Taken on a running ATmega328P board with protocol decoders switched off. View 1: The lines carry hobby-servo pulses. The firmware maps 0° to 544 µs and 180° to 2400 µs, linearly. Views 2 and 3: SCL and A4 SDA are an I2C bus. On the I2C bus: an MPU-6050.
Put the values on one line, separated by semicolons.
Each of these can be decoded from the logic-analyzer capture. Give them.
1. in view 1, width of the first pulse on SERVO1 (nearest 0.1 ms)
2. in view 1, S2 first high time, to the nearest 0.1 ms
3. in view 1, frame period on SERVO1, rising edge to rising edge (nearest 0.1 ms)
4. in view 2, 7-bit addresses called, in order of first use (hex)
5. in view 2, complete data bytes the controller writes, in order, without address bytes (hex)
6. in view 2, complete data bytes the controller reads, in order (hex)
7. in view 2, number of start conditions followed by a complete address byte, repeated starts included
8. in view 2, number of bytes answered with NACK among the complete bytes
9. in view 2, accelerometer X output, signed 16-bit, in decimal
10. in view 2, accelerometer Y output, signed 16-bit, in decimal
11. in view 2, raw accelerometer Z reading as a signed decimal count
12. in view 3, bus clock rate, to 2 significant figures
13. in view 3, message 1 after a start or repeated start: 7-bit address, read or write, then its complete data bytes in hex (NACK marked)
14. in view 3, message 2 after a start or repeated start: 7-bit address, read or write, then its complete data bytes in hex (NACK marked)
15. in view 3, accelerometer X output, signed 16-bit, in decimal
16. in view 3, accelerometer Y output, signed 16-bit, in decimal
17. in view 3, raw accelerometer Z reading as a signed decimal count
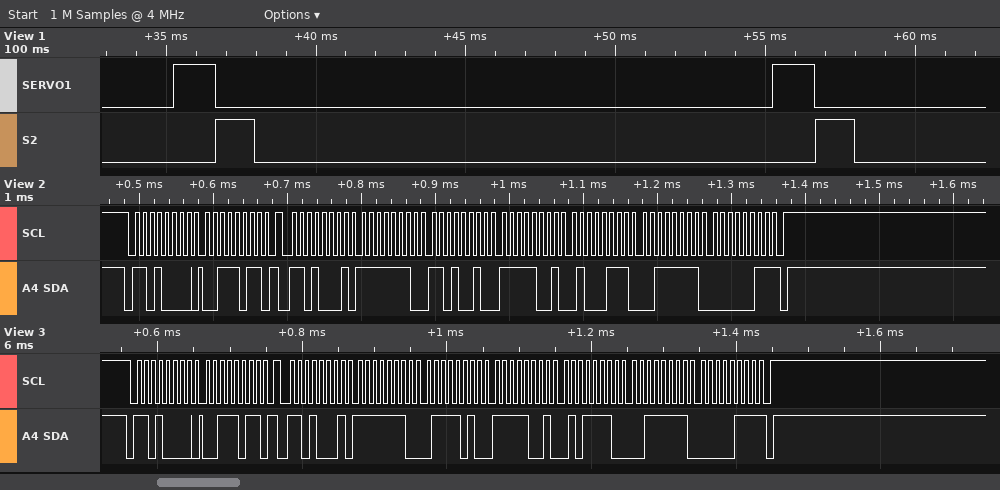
1.4 ms; 1.3 ms; 20.0 ms; 0x68; 3B; FE D2 F9 47 3F 03; 2; 1; -302; -1721; 16131; 100 kHz; 0x68 write: 3B; 0x68 read: FE 7A F9 5E 3F 07 NACK; -390; -1698; 16135
